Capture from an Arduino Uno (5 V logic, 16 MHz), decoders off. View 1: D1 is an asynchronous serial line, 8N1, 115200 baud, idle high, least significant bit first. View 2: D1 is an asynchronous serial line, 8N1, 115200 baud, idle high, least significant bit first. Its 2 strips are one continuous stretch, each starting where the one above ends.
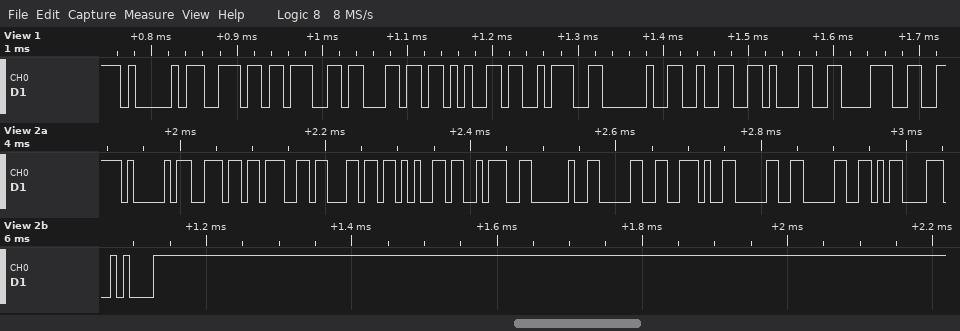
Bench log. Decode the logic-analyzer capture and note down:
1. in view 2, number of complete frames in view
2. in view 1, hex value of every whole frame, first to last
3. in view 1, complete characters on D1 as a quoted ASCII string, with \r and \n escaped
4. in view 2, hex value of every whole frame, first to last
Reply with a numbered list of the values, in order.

1. 13
2. 0x41 0x6E 0x67 0x6C 0x65 0x3A 0x20 0x32 0x31 0x38
3. "Angle: 218"
4. 41 6E 67 6C 65 3A 20 30 2E 30 30 0D 0A
